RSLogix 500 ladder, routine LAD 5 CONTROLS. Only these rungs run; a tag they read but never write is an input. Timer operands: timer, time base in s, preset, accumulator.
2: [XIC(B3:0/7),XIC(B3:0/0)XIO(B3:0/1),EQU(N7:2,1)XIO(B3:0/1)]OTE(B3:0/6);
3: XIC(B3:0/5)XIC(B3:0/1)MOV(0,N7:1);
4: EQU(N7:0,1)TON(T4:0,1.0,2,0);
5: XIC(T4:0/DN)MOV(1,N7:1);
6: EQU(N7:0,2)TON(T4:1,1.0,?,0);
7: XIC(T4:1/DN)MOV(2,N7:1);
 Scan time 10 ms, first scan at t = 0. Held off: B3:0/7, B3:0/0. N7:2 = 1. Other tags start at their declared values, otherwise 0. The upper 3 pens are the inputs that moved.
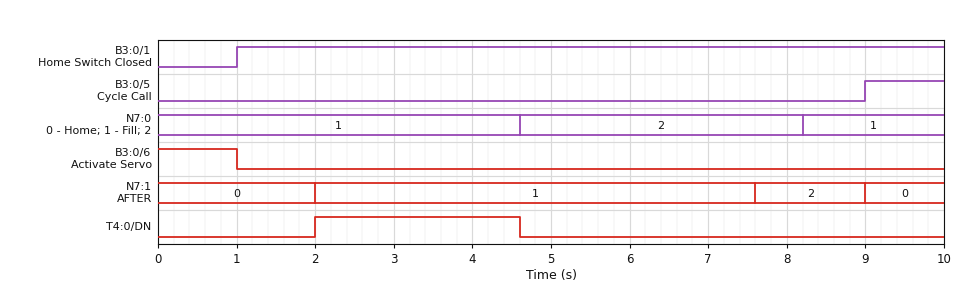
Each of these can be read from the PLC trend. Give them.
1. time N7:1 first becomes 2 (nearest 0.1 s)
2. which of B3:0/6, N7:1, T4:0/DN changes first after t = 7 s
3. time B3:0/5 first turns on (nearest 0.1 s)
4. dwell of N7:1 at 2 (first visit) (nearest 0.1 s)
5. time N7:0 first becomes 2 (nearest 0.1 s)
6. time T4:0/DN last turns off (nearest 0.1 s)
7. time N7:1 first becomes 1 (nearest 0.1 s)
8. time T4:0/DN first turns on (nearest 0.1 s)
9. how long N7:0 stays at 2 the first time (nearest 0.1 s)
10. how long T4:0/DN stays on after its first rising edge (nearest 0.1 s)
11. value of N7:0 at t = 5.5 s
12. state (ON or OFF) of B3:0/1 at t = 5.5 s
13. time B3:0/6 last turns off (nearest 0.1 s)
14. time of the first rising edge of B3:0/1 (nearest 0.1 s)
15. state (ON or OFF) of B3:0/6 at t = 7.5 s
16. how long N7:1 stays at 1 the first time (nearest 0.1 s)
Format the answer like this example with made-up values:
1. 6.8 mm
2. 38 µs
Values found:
1. 7.6 s
2. N7:1
3. 9.0 s
4. 1.4 s
5. 4.6 s
6. 4.6 s
7. 2.0 s
8. 2.0 s
9. 3.6 s
10. 2.6 s
11. 2
12. ON
13. 1.0 s
14. 1.0 s
15. OFF
16. 5.6 s
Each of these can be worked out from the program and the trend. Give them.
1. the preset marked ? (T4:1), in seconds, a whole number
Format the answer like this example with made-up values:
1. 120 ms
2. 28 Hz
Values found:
1. 3 s
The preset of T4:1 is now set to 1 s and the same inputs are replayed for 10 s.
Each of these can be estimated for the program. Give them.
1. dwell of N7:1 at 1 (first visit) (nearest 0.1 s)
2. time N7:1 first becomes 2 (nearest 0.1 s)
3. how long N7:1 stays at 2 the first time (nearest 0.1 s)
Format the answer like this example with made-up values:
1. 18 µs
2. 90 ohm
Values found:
1. 3.6 s
2. 5.6 s
3. 3.4 s
